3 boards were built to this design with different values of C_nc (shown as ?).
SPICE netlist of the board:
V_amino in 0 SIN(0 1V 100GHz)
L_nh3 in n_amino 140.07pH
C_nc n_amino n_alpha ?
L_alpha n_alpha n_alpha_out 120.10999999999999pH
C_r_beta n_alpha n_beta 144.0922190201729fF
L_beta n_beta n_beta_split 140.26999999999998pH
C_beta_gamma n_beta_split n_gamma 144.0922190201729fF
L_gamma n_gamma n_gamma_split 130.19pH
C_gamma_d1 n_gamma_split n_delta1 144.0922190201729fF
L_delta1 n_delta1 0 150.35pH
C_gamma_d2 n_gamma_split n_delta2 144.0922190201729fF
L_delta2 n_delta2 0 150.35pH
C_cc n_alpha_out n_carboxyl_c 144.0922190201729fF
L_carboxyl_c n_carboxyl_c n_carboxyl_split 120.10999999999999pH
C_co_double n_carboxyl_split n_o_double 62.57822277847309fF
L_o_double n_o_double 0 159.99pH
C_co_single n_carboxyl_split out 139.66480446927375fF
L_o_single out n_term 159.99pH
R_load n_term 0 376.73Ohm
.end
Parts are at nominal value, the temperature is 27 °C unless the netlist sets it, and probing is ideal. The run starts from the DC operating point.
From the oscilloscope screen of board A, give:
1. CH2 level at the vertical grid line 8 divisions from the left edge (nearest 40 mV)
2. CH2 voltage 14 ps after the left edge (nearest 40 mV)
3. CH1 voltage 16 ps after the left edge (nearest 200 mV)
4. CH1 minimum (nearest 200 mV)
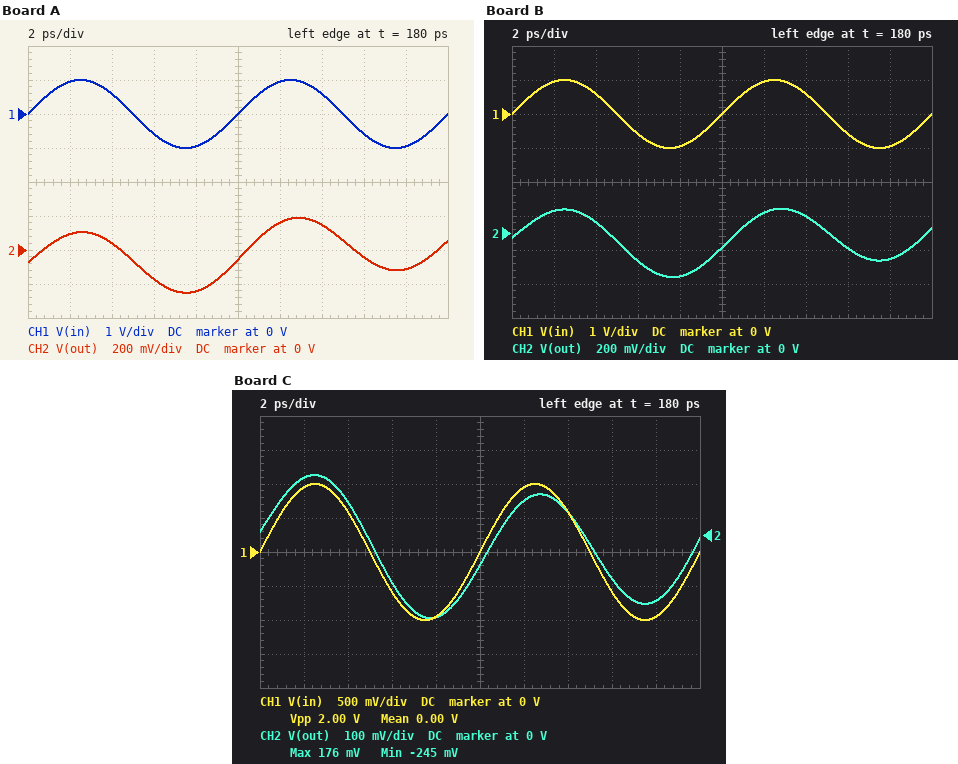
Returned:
-40 mV
160 mV
-600 mV
-1.0 V
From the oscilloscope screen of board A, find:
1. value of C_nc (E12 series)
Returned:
390 fF
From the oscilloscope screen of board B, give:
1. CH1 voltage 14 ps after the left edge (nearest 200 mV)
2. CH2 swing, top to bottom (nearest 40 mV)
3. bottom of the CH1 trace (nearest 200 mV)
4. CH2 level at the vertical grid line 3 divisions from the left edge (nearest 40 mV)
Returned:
600 mV
400 mV
-1.0 V
-160 mV
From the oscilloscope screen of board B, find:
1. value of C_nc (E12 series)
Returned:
470 fF
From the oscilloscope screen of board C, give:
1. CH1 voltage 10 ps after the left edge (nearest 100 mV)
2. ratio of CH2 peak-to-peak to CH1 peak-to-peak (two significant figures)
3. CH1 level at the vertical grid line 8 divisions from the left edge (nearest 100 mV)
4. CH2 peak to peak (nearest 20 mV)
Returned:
0 V
0.21
-600 mV
420 mV
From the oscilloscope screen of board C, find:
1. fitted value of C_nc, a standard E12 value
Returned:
560 fF
